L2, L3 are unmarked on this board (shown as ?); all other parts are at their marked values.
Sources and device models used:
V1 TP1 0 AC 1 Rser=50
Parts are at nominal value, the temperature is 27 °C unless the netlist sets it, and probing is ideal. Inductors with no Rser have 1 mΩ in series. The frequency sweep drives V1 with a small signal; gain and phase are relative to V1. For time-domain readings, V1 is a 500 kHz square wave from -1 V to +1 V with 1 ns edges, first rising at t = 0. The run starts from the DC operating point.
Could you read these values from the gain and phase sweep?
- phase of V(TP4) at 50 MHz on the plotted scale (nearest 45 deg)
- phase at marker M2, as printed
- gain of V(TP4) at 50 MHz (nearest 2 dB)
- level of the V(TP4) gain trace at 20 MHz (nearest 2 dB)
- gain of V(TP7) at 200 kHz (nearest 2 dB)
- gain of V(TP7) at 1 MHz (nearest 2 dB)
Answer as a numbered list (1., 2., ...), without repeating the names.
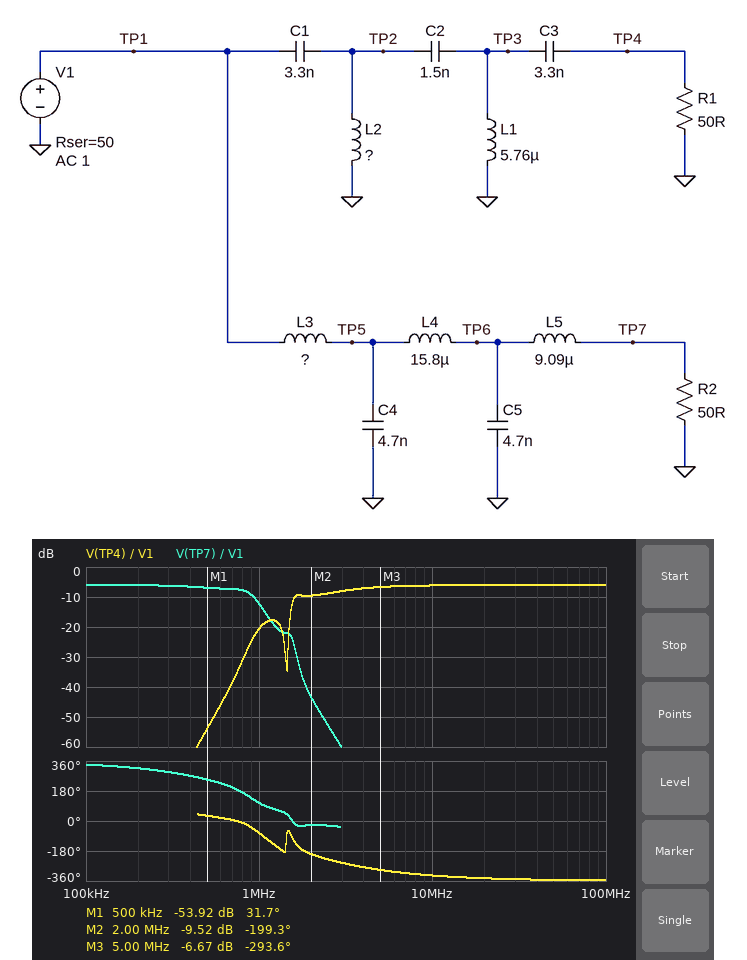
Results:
1. -360 deg
2. -199.3 deg
3. -6 dB
4. -6 dB
5. -6 dB
6. -12 dB
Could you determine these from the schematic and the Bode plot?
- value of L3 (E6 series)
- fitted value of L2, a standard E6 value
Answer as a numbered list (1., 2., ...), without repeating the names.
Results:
1. 3.3 µH
2. 2.2 µH
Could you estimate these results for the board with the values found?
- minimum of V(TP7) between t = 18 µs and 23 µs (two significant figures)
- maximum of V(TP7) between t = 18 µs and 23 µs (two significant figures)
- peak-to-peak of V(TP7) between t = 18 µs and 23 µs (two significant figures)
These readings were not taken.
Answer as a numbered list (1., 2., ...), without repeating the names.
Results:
1. -540 mV
2. 540 mV
3. 1.1 V
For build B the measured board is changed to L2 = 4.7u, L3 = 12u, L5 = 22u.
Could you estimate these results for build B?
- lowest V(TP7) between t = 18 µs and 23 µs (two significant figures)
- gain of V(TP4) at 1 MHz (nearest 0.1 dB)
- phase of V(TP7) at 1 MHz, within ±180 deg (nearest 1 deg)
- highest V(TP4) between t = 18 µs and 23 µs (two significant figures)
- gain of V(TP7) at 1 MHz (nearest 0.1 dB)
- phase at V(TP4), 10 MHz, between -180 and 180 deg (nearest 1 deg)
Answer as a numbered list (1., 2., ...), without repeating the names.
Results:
1. -570 mV
2. -13.0 dB
3. 53 deg
4. 1.1 V
5. -13.9 dB
6. 22 deg
